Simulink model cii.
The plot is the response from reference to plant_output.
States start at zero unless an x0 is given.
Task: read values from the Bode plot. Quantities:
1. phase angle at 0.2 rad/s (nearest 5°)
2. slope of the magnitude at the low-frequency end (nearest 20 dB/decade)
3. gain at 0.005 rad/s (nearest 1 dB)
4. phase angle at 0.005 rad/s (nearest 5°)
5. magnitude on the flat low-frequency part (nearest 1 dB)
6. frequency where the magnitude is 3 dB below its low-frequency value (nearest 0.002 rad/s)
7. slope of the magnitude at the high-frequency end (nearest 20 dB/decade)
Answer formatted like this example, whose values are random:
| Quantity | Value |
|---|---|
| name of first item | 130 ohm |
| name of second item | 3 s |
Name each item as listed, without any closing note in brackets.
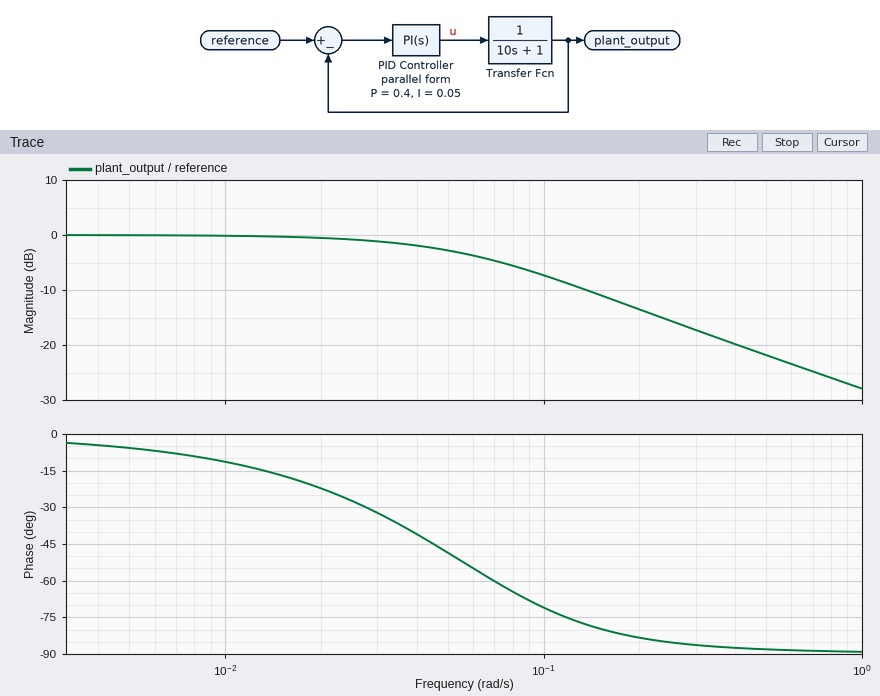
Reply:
| Quantity | Value |
|---|---|
| phase angle at 0.2 rad/s | -85° |
| slope of the magnitude at the low-frequency end | 0 dB/decade |
| gain at 0.005 rad/s | 0 dB |
| phase angle at 0.005 rad/s | -5° |
| magnitude on the flat low-frequency part | 0 dB |
| frequency where the magnitude is 3 dB below its low-frequency value | 0.052 rad/s |
| slope of the magnitude at the high-frequency end | -20 dB/decade |
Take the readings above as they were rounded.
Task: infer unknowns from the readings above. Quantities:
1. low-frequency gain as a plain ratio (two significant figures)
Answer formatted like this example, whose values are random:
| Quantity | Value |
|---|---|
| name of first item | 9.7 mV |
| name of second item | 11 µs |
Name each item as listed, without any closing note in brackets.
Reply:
| Quantity | Value |
|---|---|
| low-frequency gain as a plain ratio | 1.0 |
